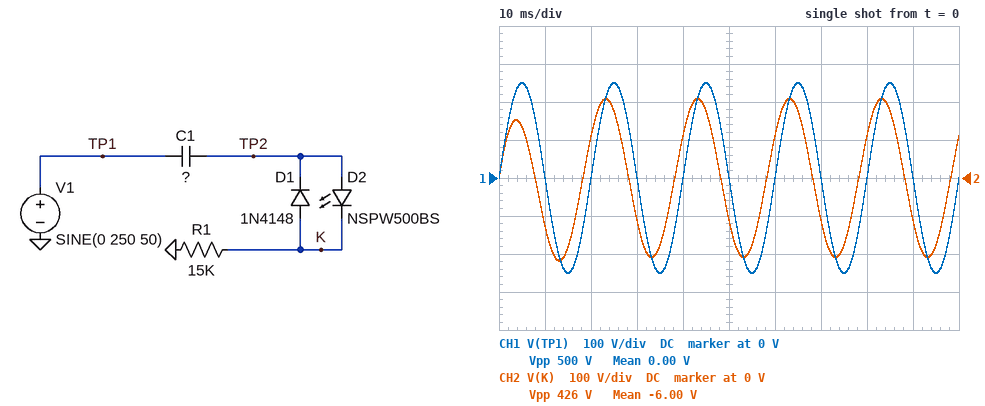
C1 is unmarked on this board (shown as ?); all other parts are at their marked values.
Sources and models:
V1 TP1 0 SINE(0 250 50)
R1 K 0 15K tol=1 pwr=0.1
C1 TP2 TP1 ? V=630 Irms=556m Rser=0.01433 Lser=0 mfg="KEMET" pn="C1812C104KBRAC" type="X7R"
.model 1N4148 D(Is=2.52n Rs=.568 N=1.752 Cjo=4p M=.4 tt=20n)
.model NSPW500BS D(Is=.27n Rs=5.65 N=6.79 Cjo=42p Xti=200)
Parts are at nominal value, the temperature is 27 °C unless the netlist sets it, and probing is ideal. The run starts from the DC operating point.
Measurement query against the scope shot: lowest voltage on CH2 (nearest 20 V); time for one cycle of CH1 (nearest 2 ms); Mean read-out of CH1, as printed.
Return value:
-220 V
20 ms
0.00 V
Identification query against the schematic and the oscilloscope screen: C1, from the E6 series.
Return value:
330 nF
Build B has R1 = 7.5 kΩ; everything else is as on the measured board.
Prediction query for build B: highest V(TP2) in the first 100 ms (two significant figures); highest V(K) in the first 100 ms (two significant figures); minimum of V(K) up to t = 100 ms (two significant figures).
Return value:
160 V
150 V
-150 V
